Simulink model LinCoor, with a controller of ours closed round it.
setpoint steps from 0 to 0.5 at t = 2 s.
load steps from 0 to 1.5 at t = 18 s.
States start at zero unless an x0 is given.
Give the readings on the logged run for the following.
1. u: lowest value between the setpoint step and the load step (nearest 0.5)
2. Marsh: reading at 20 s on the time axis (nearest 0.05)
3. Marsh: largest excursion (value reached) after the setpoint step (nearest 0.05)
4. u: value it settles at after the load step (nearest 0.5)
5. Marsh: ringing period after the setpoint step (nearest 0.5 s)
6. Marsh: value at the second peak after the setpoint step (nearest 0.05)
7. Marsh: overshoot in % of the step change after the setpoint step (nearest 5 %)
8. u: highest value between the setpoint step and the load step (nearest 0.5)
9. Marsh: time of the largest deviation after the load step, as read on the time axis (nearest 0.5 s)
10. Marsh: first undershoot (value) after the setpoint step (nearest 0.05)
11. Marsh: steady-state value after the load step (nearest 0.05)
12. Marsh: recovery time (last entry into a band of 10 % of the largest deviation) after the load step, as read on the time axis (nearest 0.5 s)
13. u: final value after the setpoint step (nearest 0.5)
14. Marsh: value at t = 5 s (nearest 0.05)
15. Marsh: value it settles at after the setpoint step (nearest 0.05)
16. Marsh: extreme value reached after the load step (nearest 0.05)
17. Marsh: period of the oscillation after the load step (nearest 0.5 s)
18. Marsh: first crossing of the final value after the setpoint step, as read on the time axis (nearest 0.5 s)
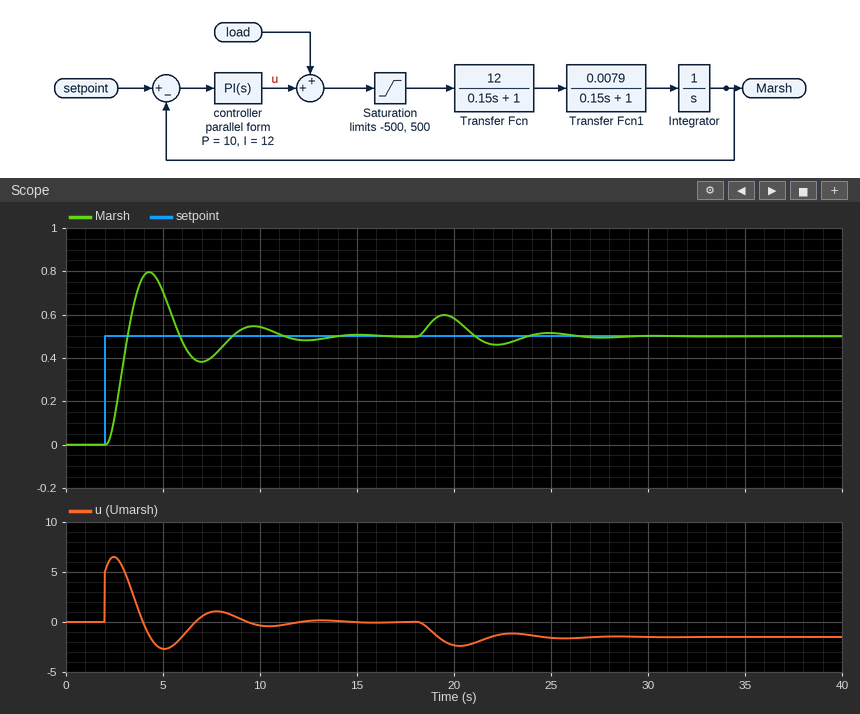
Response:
-2.5
0.60
0.80
-1.5
5.5 s
0.55
60 %
6.5
19.5 s
0.40
0.50
25.5 s
0.0
0.70
0.50
0.60
5.5 s
3.0 s
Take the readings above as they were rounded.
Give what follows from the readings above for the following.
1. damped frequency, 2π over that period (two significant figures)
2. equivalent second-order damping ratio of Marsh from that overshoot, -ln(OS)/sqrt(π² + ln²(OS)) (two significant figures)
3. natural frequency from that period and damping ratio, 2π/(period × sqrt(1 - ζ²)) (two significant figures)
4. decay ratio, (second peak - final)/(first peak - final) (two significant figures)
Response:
1.1 rad/s
0.16
1.2 rad/s
0.17
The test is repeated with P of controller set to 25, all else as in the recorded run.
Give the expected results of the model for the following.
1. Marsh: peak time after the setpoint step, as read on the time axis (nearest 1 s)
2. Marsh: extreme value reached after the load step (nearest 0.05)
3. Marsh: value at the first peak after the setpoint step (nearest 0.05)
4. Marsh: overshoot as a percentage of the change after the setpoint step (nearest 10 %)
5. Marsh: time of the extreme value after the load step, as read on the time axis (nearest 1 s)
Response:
3 s
0.55
0.70
40 %
19 s
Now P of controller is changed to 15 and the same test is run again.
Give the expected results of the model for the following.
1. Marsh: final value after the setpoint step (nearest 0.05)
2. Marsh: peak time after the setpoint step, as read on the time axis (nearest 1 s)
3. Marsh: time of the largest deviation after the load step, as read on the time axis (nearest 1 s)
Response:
0.50
4 s
19 s
